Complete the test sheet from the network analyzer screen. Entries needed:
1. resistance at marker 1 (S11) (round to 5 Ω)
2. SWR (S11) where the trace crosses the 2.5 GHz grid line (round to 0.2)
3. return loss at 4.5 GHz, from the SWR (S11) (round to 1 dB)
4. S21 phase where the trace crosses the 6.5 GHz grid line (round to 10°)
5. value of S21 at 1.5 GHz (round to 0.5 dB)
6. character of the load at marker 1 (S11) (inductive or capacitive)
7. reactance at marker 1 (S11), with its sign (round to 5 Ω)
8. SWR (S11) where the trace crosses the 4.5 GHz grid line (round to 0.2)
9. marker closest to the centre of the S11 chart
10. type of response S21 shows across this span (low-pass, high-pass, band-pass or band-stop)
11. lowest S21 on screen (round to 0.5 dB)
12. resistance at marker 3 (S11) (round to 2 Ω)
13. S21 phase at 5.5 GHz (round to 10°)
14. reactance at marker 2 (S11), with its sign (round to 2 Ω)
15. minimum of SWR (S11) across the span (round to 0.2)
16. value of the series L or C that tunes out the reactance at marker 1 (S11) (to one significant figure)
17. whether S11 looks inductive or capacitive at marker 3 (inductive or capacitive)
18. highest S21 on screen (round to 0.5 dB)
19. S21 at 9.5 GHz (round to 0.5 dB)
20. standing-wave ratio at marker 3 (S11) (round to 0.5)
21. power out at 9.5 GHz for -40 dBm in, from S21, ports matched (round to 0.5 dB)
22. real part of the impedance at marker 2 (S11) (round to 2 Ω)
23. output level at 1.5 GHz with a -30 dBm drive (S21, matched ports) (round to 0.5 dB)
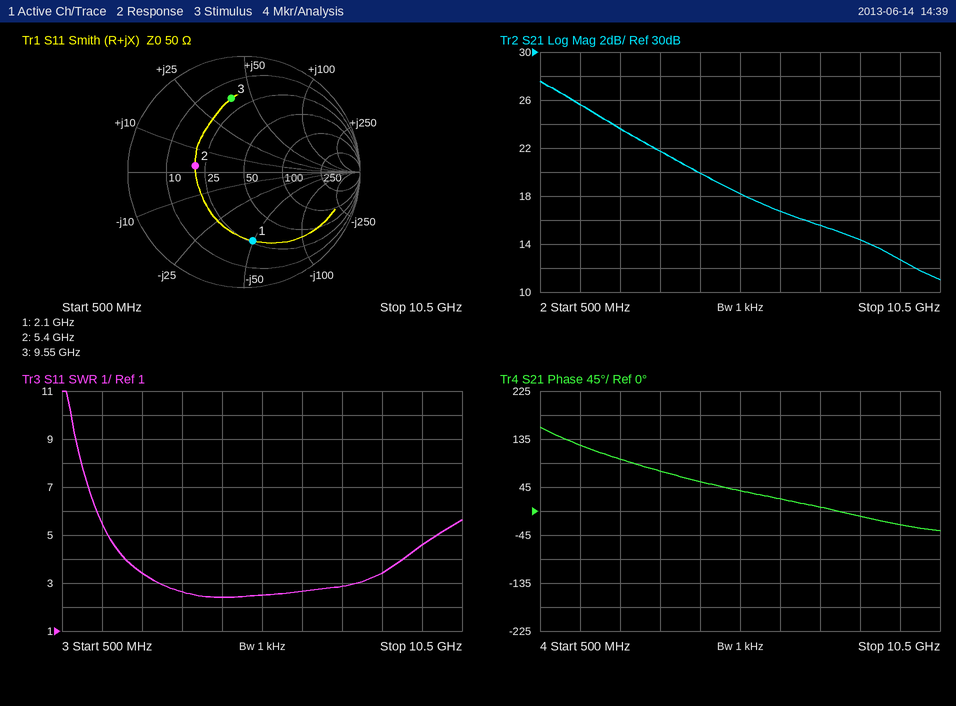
25 Ω
3.4
8 dB
20°
25.5 dB
capacitive
-50 Ω
2.4
marker 2
low-pass
11.0 dB
18 Ω
40°
+2 Ω
2.4
4 nH
inductive
27.5 dB
12.5 dB
4.5
-27.5 dBm
20 Ω
-4.5 dBm
